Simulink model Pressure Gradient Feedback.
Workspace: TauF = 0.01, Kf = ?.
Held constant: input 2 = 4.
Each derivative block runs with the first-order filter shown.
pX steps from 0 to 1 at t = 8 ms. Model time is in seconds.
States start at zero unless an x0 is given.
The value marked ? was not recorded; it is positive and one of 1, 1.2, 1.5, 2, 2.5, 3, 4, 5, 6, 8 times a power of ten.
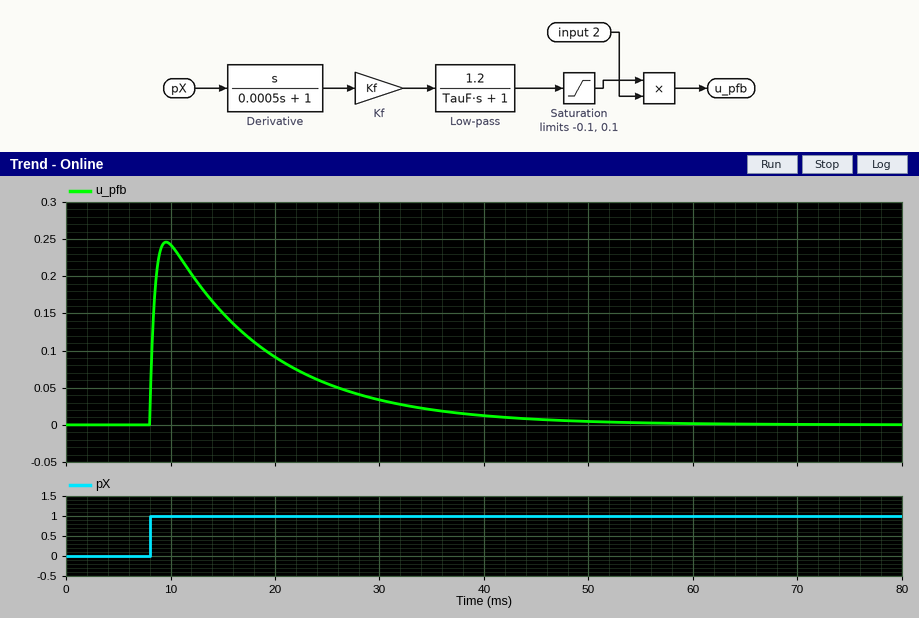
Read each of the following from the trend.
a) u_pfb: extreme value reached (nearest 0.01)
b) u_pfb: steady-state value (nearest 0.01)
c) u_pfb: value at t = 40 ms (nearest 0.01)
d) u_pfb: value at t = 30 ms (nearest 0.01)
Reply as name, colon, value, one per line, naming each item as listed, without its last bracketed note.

u_pfb: extreme value reached: 0.25
u_pfb: steady-state value: 0.00
u_pfb: value at t = 40 ms: 0.01
u_pfb: value at t = 30 ms: 0.03
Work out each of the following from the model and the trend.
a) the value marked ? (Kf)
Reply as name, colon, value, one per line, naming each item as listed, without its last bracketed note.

the value marked ?: 0.0006
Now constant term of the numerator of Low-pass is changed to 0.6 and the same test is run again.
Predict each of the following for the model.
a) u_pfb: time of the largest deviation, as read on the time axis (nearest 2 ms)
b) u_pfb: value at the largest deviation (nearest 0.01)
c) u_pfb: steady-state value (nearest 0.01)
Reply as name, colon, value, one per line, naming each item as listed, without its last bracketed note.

u_pfb: time of the largest deviation, as read on the time axis: 10 ms
u_pfb: value at the largest deviation: 0.12
u_pfb: steady-state value: 0.00
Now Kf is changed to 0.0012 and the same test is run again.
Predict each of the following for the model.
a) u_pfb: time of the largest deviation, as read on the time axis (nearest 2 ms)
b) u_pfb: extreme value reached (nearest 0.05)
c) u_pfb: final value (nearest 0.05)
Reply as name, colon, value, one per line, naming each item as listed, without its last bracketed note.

u_pfb: time of the largest deviation, as read on the time axis: 8 ms
u_pfb: extreme value reached: 0.40
u_pfb: final value: 0.00
